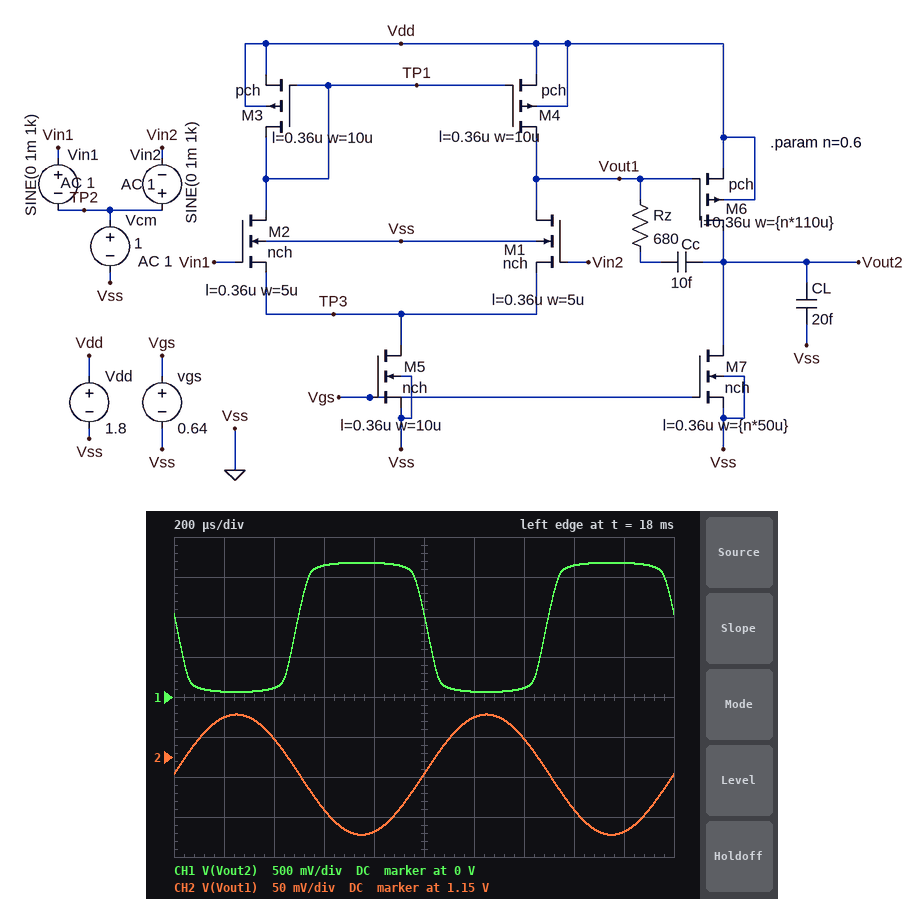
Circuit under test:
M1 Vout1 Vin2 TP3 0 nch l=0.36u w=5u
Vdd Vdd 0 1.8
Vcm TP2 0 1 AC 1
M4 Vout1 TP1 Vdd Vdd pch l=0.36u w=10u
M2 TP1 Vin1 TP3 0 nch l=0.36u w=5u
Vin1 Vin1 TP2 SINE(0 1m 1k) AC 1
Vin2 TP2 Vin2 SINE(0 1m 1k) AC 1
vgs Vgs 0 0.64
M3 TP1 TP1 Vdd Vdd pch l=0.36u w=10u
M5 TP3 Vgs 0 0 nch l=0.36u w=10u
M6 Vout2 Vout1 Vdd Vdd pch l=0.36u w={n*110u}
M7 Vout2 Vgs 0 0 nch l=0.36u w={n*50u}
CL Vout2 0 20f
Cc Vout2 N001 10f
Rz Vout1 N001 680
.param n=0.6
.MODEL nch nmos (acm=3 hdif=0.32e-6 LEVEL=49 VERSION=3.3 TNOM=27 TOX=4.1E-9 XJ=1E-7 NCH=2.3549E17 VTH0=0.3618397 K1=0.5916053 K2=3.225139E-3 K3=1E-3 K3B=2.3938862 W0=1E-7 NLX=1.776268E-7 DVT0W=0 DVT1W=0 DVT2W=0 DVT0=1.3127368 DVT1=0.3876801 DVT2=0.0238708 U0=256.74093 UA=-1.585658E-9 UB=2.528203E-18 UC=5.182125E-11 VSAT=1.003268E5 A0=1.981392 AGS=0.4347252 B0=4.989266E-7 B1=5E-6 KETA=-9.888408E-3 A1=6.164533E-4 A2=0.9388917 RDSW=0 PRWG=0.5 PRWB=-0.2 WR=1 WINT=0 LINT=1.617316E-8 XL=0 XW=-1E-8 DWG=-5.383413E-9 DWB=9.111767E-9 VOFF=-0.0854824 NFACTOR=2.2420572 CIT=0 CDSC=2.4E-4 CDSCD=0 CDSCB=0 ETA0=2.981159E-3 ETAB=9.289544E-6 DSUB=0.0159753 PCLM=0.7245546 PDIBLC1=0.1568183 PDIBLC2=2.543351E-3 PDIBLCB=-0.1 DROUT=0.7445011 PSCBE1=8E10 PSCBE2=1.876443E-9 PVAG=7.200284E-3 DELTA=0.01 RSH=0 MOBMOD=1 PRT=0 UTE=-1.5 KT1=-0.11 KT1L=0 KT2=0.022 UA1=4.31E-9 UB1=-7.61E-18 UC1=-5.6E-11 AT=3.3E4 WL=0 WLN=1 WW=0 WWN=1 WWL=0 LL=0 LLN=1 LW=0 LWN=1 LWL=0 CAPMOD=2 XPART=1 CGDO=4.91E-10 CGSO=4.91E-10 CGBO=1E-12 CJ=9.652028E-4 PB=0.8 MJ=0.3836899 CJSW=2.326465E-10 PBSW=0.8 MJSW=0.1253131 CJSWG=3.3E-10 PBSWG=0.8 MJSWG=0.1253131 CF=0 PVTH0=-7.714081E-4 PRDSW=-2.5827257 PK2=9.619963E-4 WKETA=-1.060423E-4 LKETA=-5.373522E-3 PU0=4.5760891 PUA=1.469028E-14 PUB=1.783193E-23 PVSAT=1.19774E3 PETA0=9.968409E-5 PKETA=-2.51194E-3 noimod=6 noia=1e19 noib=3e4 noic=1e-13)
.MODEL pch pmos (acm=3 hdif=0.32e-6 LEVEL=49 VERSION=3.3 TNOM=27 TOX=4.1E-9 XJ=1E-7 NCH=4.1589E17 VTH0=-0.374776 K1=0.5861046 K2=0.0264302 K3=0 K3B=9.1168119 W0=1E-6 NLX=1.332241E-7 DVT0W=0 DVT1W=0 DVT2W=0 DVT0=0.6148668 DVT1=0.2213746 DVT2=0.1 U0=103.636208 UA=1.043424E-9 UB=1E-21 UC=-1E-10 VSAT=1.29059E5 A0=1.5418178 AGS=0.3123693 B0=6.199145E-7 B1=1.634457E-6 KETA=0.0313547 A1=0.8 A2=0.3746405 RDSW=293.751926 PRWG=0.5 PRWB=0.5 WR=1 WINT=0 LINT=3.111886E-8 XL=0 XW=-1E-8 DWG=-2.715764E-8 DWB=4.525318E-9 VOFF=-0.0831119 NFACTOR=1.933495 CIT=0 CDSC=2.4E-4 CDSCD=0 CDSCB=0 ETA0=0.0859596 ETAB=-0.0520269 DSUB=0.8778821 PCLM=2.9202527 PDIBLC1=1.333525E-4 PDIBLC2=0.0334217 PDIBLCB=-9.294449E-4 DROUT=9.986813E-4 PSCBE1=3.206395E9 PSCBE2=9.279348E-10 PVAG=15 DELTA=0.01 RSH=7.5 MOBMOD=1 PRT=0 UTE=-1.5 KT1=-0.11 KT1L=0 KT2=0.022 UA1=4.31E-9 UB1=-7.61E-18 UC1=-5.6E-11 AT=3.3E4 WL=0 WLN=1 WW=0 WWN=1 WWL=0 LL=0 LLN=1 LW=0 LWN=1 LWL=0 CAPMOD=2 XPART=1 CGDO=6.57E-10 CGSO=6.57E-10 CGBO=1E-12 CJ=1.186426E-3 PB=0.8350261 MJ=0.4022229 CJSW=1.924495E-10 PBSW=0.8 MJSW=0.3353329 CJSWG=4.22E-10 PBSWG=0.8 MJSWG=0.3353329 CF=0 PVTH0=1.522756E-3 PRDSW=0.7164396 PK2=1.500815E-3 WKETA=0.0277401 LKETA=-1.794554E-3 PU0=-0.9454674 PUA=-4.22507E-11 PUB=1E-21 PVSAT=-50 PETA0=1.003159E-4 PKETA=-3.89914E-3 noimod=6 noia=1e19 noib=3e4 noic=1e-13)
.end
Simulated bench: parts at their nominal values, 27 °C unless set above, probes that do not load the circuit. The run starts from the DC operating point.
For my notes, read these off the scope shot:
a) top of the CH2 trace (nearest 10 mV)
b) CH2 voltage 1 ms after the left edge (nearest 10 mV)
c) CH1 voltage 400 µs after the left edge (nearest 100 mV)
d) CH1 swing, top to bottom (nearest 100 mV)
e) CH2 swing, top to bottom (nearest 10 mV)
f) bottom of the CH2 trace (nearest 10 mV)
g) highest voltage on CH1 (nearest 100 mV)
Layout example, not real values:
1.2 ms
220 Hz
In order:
1.20 V
1.13 V
100 mV
1.6 V
150 mV
1.05 V
1.7 V
